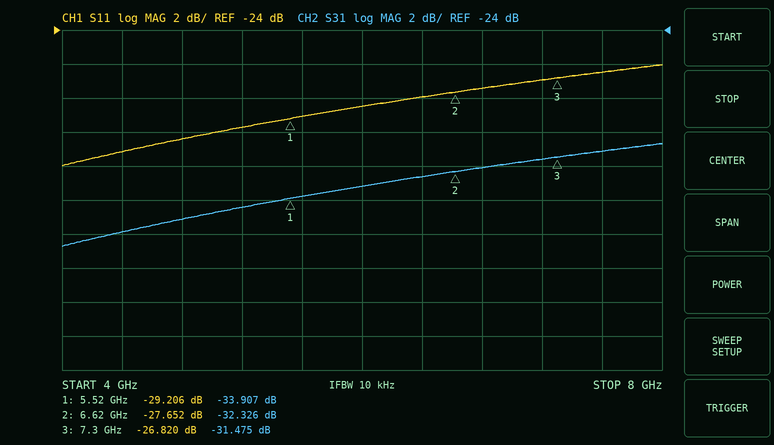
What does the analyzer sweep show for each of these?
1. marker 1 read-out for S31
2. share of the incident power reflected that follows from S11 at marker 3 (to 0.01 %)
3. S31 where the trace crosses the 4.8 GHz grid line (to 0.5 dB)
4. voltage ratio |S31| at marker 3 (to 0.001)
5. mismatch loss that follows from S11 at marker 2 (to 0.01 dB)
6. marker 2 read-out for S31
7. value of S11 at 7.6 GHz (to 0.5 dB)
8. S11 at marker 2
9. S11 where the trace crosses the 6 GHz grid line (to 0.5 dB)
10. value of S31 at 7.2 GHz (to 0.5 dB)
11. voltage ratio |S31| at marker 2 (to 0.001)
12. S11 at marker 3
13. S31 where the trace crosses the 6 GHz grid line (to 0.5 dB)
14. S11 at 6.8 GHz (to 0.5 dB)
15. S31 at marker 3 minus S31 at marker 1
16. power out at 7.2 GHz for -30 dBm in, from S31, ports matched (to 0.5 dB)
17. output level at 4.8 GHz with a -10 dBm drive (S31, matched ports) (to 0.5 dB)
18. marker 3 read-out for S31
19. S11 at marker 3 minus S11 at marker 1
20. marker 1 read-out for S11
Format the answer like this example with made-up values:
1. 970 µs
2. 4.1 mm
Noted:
1. -33.907 dB
2. 0.21 %
3. -35.0 dB
4. 0.027
5. 0.01 dB
6. -32.326 dB
7. -26.5 dB
8. -27.652 dB
9. -28.5 dB
10. -31.5 dB
11. 0.024
12. -26.820 dB
13. -33.0 dB
14. -27.5 dB
15. 2.432 dB
16. -61.5 dBm
17. -45.0 dBm
18. -31.475 dB
19. 2.386 dB
20. -29.206 dB
